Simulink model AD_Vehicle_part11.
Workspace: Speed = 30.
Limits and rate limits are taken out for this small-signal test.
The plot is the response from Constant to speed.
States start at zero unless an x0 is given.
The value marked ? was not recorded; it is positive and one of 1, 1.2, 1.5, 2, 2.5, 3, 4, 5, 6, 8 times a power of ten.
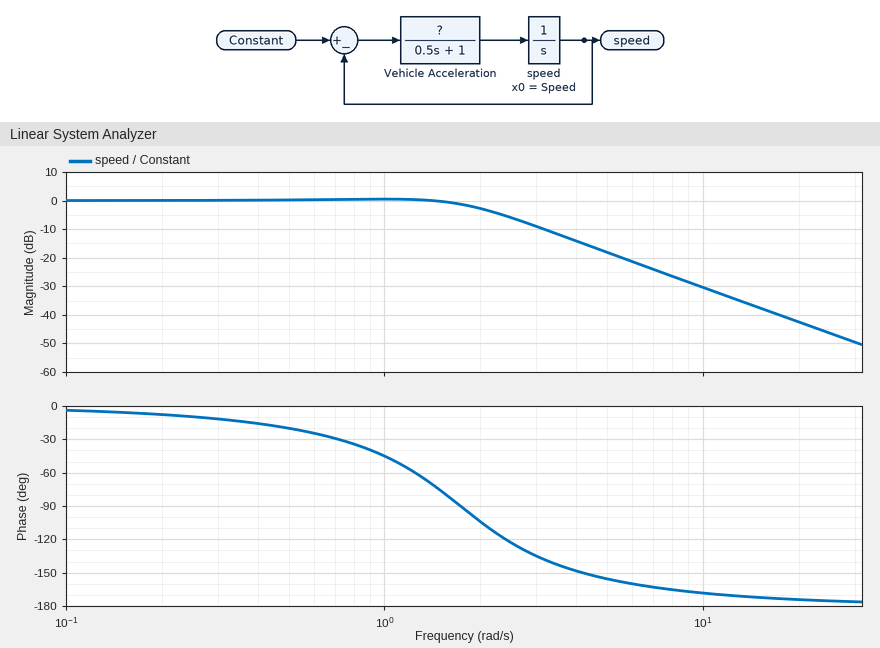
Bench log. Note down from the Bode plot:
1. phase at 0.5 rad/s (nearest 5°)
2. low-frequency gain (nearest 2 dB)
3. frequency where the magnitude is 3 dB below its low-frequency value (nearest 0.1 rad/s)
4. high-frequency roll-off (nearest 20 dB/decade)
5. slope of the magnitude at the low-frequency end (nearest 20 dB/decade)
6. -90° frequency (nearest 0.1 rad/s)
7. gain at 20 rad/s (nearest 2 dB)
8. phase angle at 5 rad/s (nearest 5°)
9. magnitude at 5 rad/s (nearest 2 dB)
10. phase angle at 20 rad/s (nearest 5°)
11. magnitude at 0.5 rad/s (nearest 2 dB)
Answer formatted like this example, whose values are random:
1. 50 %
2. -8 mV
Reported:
1. -20°
2. 0 dB
3. 2.0 rad/s
4. -40 dB/decade
5. 0 dB/decade
6. 1.7 rad/s
7. -42 dB
8. -155°
9. -18 dB
10. -175°
11. 0 dB
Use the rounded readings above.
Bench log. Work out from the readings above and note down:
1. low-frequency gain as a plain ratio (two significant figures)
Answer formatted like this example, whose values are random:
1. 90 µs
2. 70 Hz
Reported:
1. 1.0
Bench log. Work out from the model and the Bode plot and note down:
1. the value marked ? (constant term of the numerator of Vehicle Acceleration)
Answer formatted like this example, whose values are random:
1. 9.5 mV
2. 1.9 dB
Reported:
1. 1.5
